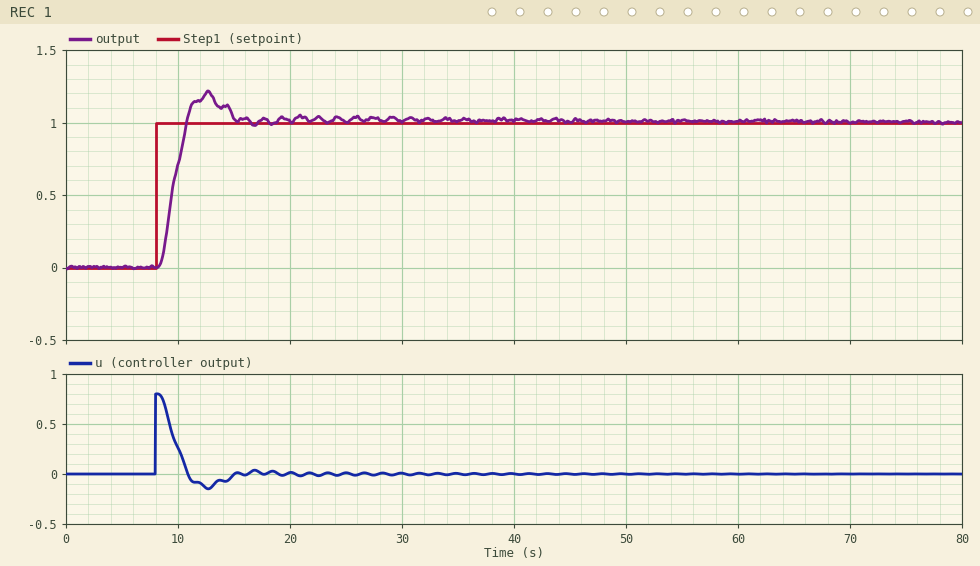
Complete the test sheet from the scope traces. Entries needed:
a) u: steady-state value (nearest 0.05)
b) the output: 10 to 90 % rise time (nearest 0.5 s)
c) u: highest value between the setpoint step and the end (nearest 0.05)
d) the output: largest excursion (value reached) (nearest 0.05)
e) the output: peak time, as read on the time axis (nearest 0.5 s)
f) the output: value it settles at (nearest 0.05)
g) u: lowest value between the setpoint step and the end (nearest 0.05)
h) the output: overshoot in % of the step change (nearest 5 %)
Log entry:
0.00
2.0 s
0.80
1.20
12.5 s
1.00
-0.15
20 %
